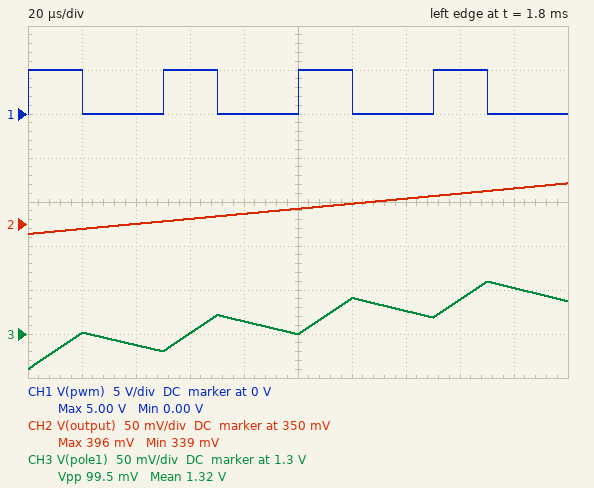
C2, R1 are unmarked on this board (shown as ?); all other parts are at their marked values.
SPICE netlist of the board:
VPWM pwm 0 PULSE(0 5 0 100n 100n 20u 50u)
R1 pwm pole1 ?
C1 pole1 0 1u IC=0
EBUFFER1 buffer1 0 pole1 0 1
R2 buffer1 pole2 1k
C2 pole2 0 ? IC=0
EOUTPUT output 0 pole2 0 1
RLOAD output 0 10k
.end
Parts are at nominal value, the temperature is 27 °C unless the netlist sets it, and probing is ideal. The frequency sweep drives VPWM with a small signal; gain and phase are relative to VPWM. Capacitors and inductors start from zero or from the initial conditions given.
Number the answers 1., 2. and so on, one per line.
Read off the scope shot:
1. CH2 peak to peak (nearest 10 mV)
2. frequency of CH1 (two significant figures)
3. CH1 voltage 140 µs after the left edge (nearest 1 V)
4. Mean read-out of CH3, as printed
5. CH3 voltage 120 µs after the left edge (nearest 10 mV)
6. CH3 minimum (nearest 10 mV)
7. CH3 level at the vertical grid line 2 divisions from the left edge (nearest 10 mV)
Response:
1. 60 mV
2. 20 kHz
3. 0 V
4. 1.32 V
5. 1.34 V
6. 1.26 V
7. 1.29 V
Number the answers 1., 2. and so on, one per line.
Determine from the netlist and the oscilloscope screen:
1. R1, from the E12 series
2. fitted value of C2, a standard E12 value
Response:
1. 1.8 kΩ
2. 3.3 µF
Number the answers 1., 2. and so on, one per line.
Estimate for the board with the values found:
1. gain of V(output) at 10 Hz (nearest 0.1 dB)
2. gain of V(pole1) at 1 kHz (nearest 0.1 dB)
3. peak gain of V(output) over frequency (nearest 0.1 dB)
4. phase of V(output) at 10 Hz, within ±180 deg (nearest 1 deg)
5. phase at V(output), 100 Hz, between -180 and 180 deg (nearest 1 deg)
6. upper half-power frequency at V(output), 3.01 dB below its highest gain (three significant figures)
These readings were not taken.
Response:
1. -0.2 dB
2. -21.1 dB
3. 0 dB
4. -18 deg
5. -113 deg
6. 39.4 Hz
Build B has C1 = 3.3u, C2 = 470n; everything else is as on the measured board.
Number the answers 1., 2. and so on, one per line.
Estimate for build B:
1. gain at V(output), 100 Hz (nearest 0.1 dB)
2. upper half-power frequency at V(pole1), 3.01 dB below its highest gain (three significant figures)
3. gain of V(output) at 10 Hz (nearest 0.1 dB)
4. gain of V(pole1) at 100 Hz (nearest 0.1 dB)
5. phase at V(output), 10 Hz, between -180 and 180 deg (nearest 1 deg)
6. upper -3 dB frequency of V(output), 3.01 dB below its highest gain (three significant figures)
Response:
1. -12.1 dB
2. 26.8 Hz
3. -0.6 dB
4. -11.7 dB
5. -22 deg
6. 26.6 Hz
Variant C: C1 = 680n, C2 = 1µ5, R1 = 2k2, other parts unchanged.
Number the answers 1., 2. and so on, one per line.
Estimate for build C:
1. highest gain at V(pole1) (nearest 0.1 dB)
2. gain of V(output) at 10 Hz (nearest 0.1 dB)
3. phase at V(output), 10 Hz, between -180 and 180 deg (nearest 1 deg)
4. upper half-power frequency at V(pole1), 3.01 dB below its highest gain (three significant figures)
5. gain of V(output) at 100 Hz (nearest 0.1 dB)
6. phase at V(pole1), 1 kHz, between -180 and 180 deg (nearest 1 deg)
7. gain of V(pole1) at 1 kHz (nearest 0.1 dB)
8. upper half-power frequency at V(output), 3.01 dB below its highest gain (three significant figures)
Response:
1. 0 dB
2. -0.1 dB
3. -11 deg
4. 106 Hz
5. -5.5 dB
6. -84 deg
7. -19.5 dB
8. 68.4 Hz
